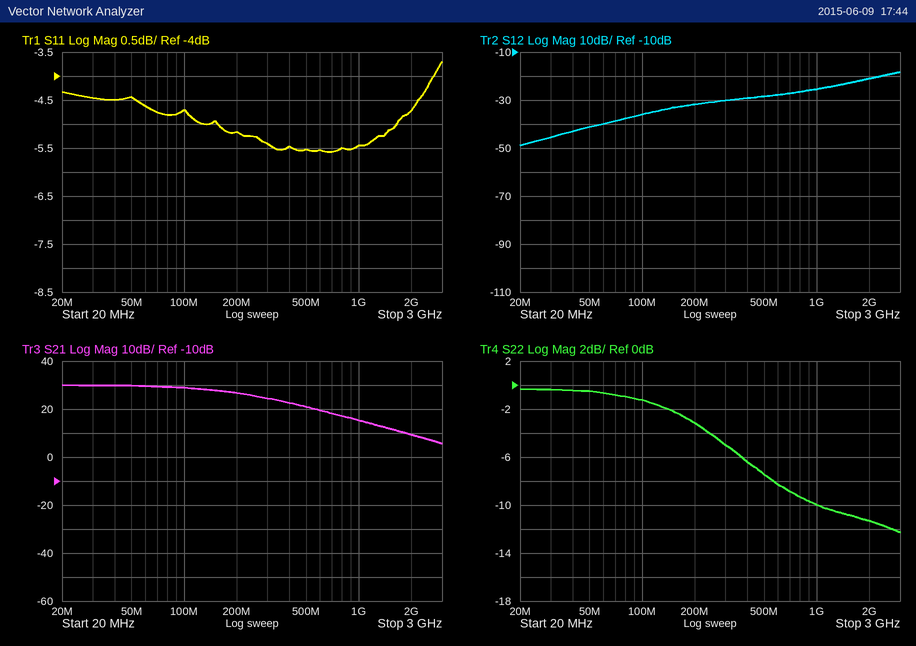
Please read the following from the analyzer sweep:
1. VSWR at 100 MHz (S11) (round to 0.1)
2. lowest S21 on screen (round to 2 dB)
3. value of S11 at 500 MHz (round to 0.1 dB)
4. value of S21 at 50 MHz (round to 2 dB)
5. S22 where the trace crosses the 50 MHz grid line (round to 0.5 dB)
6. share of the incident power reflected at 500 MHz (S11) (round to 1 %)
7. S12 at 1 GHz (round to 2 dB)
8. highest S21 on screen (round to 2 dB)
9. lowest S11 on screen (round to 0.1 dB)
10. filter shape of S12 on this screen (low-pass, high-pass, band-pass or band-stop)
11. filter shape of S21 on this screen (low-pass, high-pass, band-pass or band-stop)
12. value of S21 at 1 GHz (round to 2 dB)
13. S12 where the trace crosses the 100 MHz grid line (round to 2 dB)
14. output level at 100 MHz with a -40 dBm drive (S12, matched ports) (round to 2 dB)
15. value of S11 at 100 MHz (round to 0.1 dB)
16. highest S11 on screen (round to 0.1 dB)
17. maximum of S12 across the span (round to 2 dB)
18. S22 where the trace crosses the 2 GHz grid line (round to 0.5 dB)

3.8
6 dB
-5.5 dB
30 dB
-0.5 dB
28 %
-26 dB
30 dB
-5.6 dB
high-pass
low-pass
16 dB
-36 dB
-76 dBm
-4.7 dB
-3.7 dB
-18 dB
-11.5 dB
